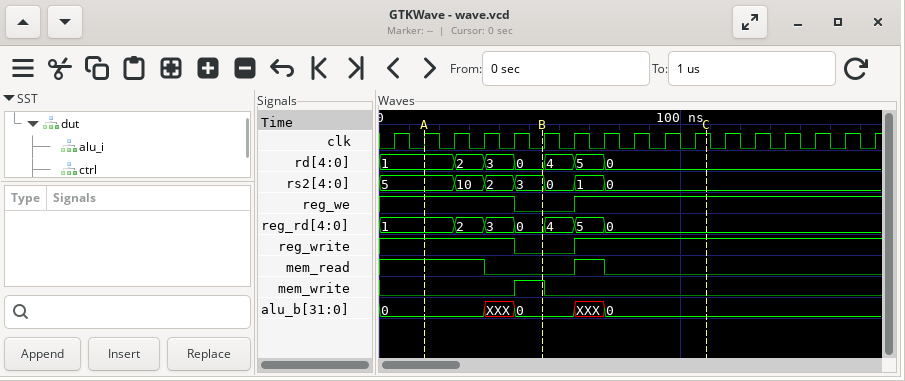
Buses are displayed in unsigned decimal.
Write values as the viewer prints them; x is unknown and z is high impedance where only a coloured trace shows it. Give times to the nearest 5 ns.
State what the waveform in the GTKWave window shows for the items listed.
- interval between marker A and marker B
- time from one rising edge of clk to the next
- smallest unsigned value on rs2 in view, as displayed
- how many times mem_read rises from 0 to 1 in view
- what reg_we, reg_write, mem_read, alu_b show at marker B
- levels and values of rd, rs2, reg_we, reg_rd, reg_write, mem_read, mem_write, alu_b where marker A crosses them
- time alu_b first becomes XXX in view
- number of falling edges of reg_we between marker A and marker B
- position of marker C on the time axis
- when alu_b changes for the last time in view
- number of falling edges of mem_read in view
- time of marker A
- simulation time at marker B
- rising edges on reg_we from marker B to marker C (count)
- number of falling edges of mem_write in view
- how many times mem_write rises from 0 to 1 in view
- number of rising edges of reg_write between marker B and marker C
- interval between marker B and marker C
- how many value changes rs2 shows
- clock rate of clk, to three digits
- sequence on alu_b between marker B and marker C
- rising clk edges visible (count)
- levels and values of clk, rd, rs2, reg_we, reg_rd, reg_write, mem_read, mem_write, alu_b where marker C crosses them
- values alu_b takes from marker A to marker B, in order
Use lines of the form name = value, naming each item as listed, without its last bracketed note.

interval between marker A and marker B = 40 ns
time from one rising edge of clk to the next = 10 ns
smallest unsigned value on rs2 in view, as displayed = 0
how many times mem_read rises from 0 to 1 in view = 1
what reg_we, reg_write, mem_read, alu_b show at marker B = reg_we=0, reg_write=0, mem_read=0, alu_b=0
levels and values of rd, rs2, reg_we, reg_rd, reg_write, mem_read, mem_write, alu_b where marker A crosses them = rd=1, rs2=5, reg_we=1, reg_rd=1, reg_write=1, mem_read=1, mem_write=0, alu_b=0
time alu_b first becomes XXX in view = 35 ns
number of falling edges of reg_we between marker A and marker B = 1
position of marker C on the time axis = 110 ns
when alu_b changes for the last time in view = 75 ns
number of falling edges of mem_read in view = 2
time of marker A = 15 ns
simulation time at marker B = 55 ns
rising edges on reg_we from marker B to marker C = 1
number of falling edges of mem_write in view = 1
how many times mem_write rises from 0 to 1 in view = 1
number of rising edges of reg_write between marker B and marker C = 1
interval between marker B and marker C = 55 ns
how many value changes rs2 shows = 6
clock rate of clk, to three digits = 100 MHz
sequence on alu_b between marker B and marker C = 0, XXX, 0
rising clk edges visible = 17
levels and values of clk, rd, rs2, reg_we, reg_rd, reg_write, mem_read, mem_write, alu_b where marker C crosses them = clk=1, rd=0, rs2=0, reg_we=1, reg_rd=0, reg_write=1, mem_read=0, mem_write=0, alu_b=0
values alu_b takes from marker A to marker B, in order = 0, XXX, 0
